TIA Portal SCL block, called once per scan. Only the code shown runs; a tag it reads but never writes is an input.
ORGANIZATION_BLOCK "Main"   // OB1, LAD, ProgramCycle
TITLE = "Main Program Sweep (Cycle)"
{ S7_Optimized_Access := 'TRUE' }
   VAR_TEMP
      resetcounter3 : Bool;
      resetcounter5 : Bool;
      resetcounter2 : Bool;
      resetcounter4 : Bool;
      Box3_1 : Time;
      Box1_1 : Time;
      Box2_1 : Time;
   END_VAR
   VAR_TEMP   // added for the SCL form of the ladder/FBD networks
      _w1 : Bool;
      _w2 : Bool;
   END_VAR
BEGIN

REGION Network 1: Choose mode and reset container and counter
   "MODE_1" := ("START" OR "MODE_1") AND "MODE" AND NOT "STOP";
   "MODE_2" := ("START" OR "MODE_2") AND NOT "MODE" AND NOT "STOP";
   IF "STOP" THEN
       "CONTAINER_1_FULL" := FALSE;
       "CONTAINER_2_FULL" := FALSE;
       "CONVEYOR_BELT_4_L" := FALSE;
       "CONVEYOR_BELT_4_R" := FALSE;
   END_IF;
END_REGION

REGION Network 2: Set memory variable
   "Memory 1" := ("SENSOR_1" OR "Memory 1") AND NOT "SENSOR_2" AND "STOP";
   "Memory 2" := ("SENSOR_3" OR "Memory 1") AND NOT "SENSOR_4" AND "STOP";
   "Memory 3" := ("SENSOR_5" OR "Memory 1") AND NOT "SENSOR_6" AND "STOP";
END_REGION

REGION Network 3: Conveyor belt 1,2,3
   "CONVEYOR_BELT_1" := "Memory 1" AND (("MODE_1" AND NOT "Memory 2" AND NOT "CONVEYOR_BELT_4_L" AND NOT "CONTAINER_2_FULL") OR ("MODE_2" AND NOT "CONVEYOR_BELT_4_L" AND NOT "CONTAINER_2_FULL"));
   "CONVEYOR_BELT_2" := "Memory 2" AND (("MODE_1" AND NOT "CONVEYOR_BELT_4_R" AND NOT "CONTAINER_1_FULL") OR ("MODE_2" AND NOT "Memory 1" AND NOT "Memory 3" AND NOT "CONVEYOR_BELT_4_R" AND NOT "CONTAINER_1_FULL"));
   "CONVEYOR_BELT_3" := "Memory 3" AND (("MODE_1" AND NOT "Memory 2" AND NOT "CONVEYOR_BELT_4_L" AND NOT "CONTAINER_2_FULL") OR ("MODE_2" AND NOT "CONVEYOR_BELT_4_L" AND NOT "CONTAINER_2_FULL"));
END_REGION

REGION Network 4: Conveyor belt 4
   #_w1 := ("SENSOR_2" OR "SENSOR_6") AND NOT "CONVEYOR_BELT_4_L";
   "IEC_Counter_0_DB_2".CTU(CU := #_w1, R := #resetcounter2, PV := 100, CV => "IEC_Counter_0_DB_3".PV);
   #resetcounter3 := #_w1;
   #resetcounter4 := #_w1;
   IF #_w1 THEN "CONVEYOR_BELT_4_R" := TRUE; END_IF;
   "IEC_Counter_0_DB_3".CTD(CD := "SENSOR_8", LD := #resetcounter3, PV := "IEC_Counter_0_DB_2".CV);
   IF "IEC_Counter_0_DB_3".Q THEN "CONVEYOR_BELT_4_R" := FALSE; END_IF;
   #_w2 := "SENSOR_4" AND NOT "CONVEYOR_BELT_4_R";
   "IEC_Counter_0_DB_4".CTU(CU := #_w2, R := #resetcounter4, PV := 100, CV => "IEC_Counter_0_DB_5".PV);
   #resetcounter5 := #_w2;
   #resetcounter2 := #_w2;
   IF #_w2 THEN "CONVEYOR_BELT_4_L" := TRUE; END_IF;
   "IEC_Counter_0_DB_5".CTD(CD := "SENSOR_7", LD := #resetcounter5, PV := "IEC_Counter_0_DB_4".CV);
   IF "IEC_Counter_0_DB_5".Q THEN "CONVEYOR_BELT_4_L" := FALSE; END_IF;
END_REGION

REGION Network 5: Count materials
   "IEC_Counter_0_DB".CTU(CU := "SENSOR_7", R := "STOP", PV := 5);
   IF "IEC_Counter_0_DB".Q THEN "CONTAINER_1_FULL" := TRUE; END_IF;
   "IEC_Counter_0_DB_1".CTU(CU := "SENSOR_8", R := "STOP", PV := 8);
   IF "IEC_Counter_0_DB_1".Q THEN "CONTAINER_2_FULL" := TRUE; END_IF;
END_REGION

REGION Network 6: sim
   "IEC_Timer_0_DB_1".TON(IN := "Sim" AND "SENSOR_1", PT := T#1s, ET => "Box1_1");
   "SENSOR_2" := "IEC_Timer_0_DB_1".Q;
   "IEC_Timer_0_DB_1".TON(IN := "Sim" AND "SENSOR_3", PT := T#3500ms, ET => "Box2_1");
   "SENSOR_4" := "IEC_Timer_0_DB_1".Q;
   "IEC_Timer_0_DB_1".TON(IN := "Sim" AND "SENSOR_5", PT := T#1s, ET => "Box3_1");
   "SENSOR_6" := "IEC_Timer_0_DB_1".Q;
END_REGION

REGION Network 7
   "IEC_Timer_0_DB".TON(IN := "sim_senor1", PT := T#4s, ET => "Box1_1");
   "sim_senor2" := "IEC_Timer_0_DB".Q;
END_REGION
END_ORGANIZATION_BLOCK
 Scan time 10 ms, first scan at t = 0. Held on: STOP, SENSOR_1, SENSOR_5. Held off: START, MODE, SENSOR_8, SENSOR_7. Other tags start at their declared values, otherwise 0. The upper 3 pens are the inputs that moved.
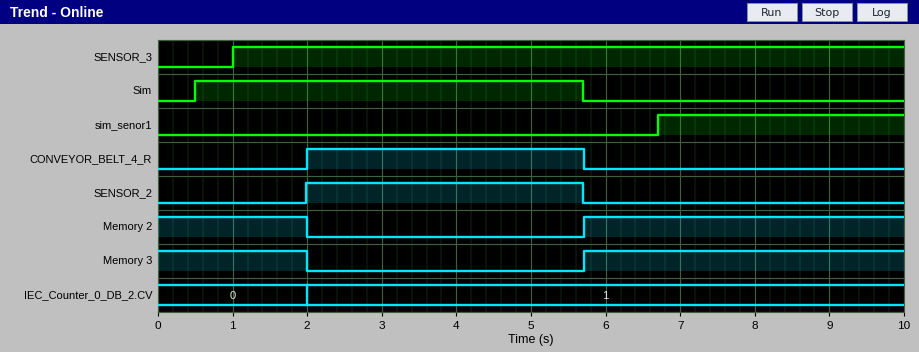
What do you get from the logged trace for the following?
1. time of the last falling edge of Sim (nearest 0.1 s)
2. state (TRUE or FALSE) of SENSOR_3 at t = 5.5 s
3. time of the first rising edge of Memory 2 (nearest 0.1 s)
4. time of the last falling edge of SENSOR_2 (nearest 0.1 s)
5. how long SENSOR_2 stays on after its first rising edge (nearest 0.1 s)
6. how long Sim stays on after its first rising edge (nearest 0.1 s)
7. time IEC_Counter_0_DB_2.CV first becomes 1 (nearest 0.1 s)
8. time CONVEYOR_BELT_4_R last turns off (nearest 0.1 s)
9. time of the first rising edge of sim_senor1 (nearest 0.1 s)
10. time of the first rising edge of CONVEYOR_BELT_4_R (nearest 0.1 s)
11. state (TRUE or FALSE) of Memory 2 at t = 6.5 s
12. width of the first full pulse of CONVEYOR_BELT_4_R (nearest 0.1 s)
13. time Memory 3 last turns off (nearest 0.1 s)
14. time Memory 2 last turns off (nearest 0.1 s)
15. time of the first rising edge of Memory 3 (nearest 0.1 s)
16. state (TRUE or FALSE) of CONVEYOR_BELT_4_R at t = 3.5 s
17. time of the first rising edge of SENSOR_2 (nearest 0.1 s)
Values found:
5.7 s
TRUE
5.7 s
5.7 s
3.7 s
5.2 s
2.0 s
5.7 s
6.7 s
2.0 s
TRUE
3.7 s
2.0 s
2.0 s
5.7 s
TRUE
2.0 s
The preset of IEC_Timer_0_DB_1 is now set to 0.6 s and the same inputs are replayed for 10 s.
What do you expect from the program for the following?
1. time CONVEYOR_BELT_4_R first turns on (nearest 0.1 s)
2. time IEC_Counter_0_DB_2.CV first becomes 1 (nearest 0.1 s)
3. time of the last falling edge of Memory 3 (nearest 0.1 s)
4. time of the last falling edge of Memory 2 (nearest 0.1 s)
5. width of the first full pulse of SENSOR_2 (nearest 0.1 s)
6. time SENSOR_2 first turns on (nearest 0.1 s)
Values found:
1.6 s
1.6 s
1.6 s
1.6 s
4.1 s
1.6 s
